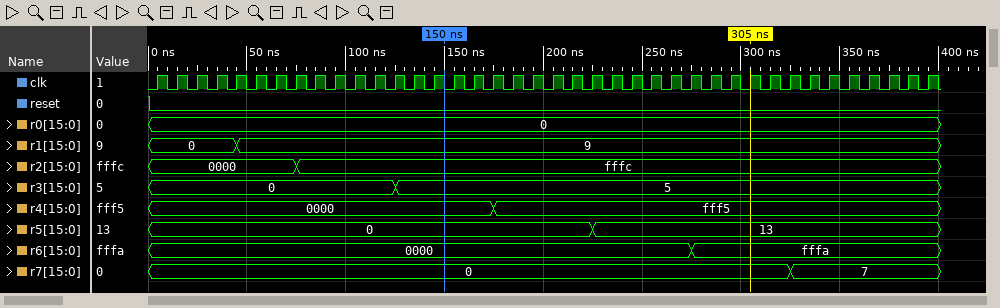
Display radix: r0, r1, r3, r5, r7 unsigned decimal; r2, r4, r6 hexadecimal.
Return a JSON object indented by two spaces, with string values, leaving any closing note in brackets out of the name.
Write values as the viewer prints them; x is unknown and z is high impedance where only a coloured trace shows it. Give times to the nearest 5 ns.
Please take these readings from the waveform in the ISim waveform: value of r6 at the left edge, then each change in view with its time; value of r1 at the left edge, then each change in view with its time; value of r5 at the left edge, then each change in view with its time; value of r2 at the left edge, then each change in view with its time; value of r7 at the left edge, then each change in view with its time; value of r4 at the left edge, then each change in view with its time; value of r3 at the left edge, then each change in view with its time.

{
  "value of r6 at the left edge, then each change in view with its time": "0000, fffa at 275 ns",
  "value of r1 at the left edge, then each change in view with its time": "0, 9 at 45 ns",
  "value of r5 at the left edge, then each change in view with its time": "0, 13 at 225 ns",
  "value of r2 at the left edge, then each change in view with its time": "0000, fffc at 75 ns",
  "value of r7 at the left edge, then each change in view with its time": "0, 7 at 325 ns",
  "value of r4 at the left edge, then each change in view with its time": "0000, fff5 at 175 ns",
  "value of r3 at the left edge, then each change in view with its time": "0, 5 at 125 ns"
}
